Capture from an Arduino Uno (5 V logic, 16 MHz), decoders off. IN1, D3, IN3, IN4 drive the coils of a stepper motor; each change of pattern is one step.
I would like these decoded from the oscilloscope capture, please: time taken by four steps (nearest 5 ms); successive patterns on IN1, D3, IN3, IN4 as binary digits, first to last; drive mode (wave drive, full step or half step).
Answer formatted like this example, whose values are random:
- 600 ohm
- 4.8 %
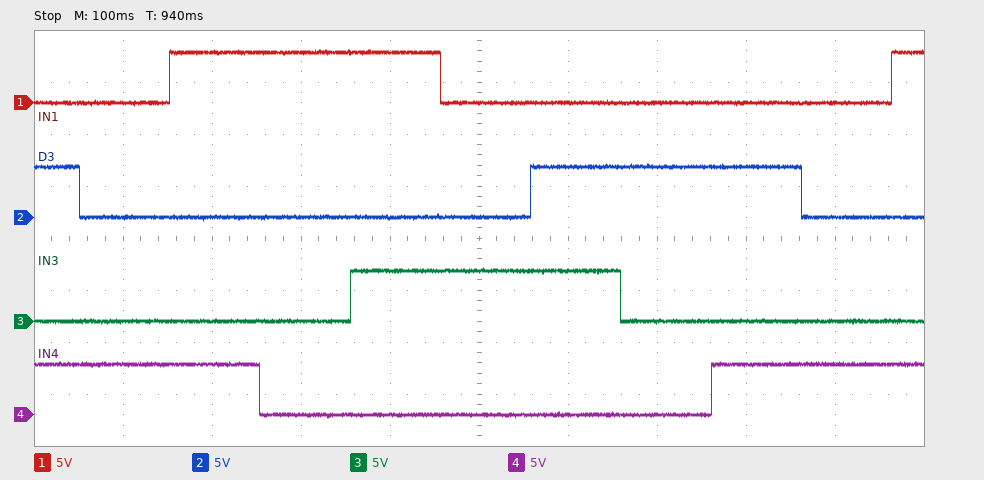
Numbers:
- 405 ms
- 0101 0001 1001 1000 1010 0010 0110 0100 0101 0001 1001
- half step
